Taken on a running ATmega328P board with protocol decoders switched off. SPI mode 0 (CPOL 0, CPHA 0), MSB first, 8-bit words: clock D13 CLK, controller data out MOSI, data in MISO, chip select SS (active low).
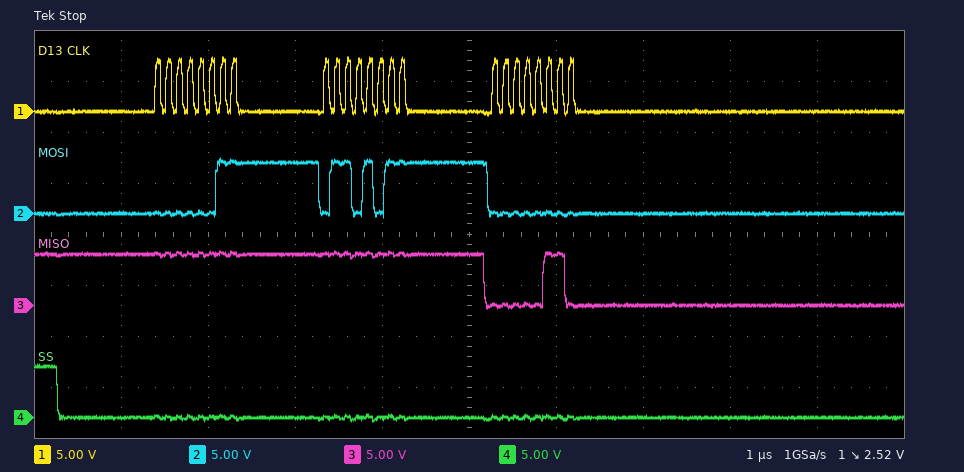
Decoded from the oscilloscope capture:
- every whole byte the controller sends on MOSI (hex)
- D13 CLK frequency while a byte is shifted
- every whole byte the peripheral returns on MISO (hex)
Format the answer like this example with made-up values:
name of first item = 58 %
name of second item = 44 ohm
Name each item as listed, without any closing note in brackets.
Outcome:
every whole byte the controller sends on MOSI = 03 6B 00
D13 CLK frequency while a byte is shifted = 8 MHz
every whole byte the peripheral returns on MISO = FF FF 06
